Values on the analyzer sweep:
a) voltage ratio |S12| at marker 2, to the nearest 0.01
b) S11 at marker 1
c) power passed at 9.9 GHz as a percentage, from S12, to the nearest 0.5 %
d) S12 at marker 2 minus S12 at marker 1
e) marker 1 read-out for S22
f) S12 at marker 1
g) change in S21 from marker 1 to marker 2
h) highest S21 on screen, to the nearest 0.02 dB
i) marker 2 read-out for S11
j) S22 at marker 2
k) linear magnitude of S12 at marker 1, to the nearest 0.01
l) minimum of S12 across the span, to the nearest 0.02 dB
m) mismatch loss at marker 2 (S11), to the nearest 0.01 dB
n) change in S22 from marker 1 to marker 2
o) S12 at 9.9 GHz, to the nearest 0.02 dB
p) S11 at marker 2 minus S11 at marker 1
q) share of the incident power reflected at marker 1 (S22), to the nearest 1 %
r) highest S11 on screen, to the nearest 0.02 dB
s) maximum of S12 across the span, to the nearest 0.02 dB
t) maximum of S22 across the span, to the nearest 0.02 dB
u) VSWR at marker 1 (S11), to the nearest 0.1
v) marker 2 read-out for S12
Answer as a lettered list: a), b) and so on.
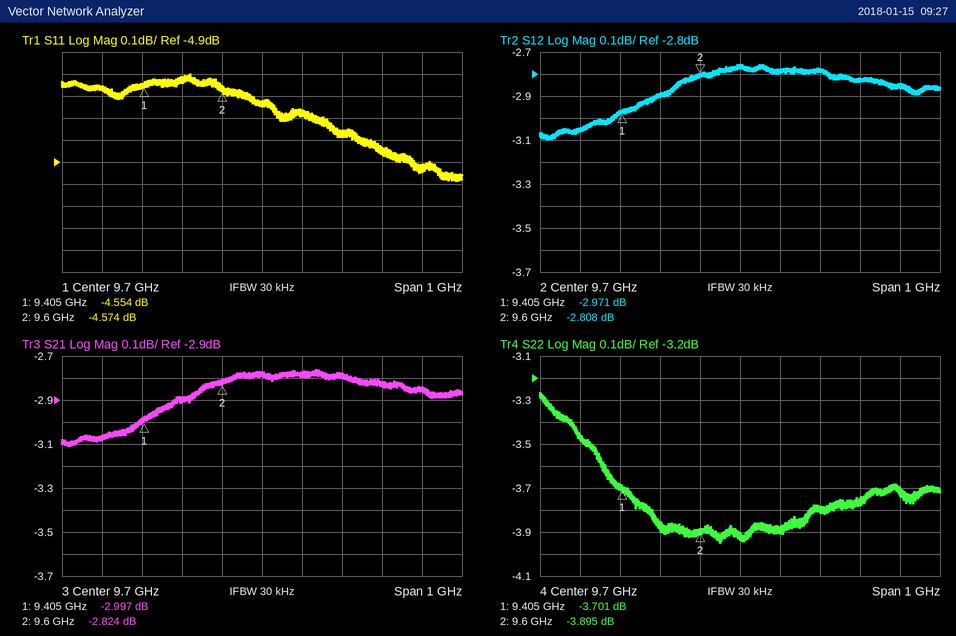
a) 0.72
b) -4.554 dB
c) 52.5 %
d) 0.163 dB
e) -3.701 dB
f) -2.971 dB
g) 0.173 dB
h) -2.76 dB
i) -4.574 dB
j) -3.895 dB
k) 0.71
l) -3.10 dB
m) 1.86 dB
n) -0.194 dB
o) -2.78 dB
p) -0.020 dB
q) 43 %
r) -4.50 dB
s) -2.76 dB
t) -3.26 dB
u) 3.9
v) -2.808 dB
